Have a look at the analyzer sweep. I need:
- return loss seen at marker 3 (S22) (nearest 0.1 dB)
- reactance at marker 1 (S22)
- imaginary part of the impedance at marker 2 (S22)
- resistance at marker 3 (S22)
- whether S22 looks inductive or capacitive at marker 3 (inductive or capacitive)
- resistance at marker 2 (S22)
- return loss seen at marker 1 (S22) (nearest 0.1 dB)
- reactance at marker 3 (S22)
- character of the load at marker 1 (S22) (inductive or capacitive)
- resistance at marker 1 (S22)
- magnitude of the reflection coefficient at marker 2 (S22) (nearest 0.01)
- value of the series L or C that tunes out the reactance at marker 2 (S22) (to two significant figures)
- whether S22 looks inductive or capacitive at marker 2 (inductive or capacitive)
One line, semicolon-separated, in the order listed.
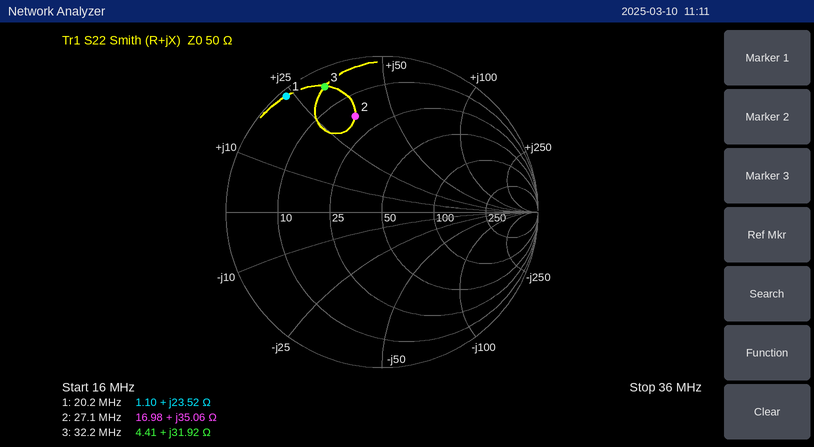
1.1 dB; +23.52 Ω; +35.06 Ω; 4.41 Ω; inductive; 16.98 Ω; 0.3 dB; +31.92 Ω; inductive; 1.10 Ω; 0.64; 170 pF; inductive
